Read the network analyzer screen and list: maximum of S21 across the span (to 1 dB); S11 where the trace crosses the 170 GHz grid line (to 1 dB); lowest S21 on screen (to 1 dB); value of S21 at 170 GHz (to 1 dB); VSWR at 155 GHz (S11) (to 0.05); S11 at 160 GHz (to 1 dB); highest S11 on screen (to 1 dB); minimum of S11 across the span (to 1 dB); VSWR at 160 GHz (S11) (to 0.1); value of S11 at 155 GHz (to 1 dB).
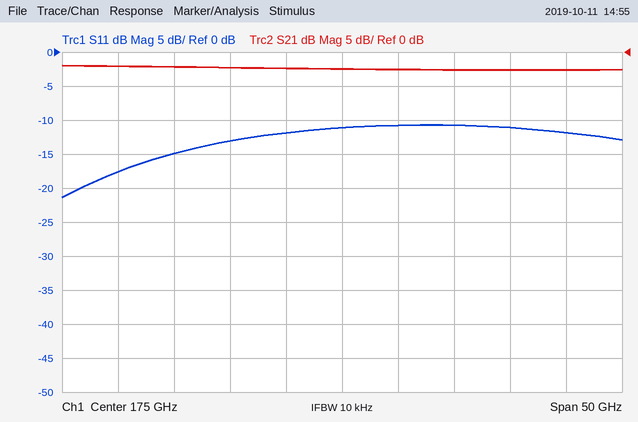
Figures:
-2 dB
-12 dB
-3 dB
-2 dB
1.30
-15 dB
-11 dB
-21 dB
1.4
-18 dB
